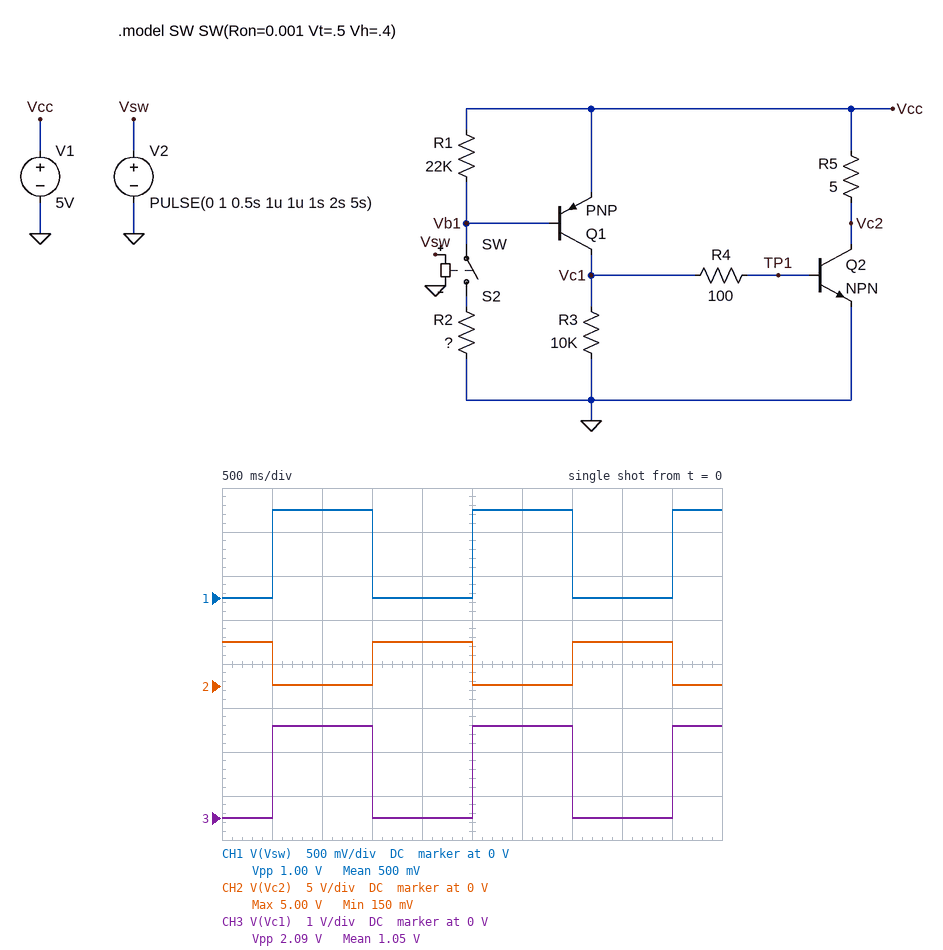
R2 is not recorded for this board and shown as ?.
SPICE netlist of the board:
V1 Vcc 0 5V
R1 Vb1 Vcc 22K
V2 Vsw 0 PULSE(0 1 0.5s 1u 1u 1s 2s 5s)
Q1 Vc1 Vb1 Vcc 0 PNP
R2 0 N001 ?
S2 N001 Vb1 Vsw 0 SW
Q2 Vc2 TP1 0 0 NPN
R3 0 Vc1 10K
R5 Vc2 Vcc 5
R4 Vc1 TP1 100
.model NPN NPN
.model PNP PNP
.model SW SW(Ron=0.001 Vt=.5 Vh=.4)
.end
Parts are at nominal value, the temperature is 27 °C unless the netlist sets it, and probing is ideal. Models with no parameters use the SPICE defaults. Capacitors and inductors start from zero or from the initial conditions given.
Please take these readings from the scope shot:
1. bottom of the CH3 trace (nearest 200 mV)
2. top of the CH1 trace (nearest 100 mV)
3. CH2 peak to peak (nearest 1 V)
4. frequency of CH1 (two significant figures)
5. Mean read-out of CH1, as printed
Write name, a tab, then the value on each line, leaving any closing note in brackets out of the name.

bottom of the CH3 trace	0 V
top of the CH1 trace	1.0 V
CH2 peak to peak	5 V
frequency of CH1	500 mHz
Mean read-out of CH1, as printed	500 mV
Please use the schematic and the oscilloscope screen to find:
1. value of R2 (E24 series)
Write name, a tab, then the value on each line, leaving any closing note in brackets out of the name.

value of R2	27 kΩ
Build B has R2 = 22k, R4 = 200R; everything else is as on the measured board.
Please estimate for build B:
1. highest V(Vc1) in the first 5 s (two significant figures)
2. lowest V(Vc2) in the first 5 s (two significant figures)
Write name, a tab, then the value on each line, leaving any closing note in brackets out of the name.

highest V(Vc1) in the first 5 s	3.9 V
lowest V(Vc2) in the first 5 s	140 mV
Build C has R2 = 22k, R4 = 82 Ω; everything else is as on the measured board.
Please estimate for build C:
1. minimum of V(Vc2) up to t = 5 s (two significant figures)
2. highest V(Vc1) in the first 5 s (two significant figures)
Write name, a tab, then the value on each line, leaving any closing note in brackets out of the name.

minimum of V(Vc2) up to t = 5 s	140 mV
highest V(Vc1) in the first 5 s	2.2 V
